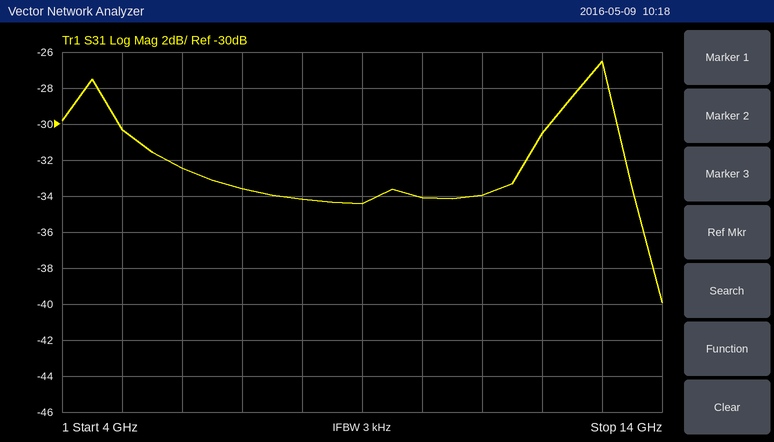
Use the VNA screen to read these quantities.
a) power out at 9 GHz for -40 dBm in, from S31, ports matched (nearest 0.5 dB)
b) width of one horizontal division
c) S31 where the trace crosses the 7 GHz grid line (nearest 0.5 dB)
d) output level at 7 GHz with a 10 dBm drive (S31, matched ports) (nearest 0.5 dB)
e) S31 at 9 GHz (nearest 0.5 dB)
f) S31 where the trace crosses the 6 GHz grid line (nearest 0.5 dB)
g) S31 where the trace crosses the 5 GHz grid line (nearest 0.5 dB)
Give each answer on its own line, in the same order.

-74.5 dBm
1 GHz
-33.5 dB
-23.5 dBm
-34.5 dB
-32.5 dB
-30.5 dB
